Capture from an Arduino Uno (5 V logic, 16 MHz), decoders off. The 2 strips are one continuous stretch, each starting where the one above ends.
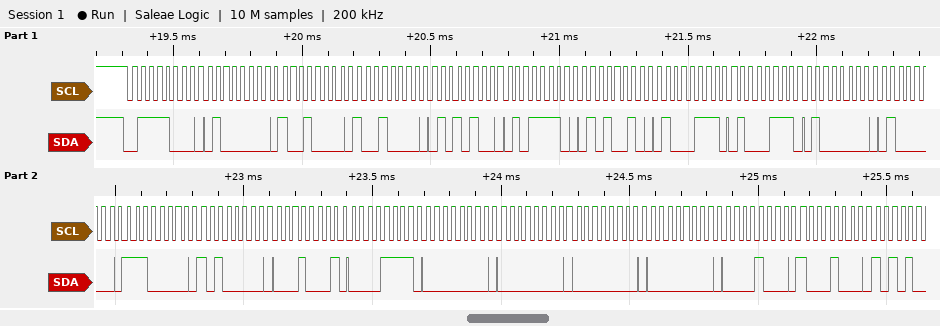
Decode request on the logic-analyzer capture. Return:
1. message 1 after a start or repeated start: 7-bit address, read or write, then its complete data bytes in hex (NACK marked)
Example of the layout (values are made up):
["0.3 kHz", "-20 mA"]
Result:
["0x3C write: 40 90 90 54 5E 52 47 47 40 40 E0 A0 11 0F 00 00 00 00 08 88"]
